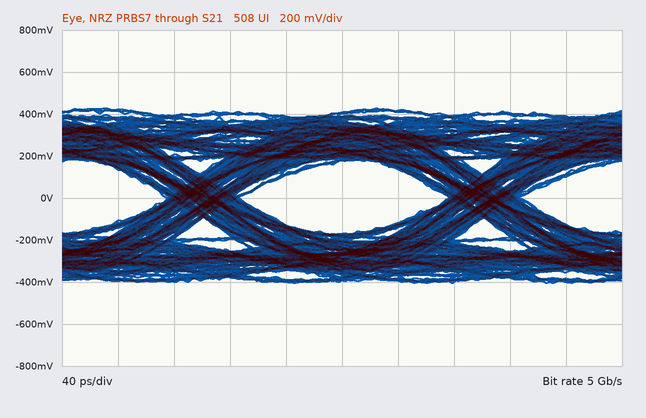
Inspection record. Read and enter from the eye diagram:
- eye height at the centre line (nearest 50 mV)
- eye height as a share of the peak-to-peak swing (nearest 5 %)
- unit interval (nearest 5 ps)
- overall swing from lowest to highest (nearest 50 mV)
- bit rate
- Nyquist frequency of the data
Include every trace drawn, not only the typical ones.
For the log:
350 mV
40 %
200 ps
850 mV
5 Gb/s
2.5 GHz
